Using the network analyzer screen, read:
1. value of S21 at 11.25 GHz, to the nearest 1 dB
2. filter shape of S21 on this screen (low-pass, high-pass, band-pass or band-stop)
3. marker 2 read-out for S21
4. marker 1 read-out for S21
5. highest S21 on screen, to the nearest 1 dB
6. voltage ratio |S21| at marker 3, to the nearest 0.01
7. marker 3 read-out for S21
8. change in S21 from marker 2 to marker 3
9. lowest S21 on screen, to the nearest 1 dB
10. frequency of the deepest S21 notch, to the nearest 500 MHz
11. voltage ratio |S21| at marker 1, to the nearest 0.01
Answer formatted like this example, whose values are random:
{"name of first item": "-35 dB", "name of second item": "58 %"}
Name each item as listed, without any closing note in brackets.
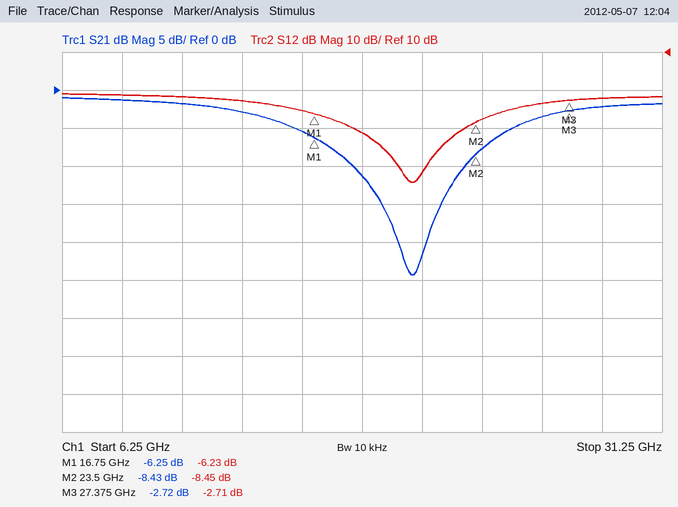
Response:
{"value of S21 at 11.25 GHz, to the nearest 1 dB": "-2 dB", "filter shape of S21 on this screen": "band-stop", "marker 2 read-out for S21": "-8.43 dB", "marker 1 read-out for S21": "-6.25 dB", "highest S21 on screen, to the nearest 1 dB": "-1 dB", "voltage ratio |S21| at marker 3, to the nearest 0.01": "0.73", "marker 3 read-out for S21": "-2.72 dB", "change in S21 from marker 2 to marker 3": "5.71 dB", "lowest S21 on screen, to the nearest 1 dB": "-24 dB", "frequency of the deepest S21 notch, to the nearest 500 MHz": "21.0 GHz", "voltage ratio |S21| at marker 1, to the nearest 0.01": "0.49"}
